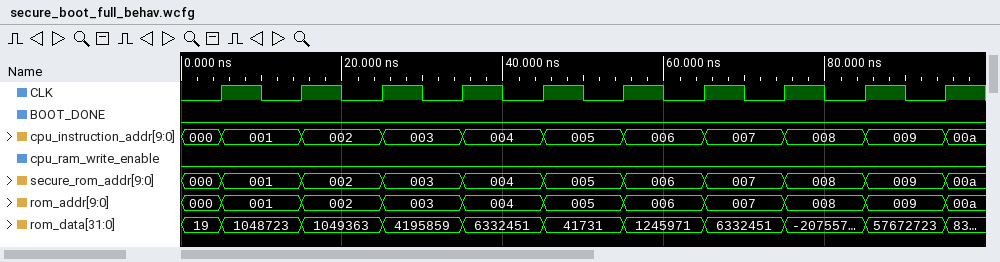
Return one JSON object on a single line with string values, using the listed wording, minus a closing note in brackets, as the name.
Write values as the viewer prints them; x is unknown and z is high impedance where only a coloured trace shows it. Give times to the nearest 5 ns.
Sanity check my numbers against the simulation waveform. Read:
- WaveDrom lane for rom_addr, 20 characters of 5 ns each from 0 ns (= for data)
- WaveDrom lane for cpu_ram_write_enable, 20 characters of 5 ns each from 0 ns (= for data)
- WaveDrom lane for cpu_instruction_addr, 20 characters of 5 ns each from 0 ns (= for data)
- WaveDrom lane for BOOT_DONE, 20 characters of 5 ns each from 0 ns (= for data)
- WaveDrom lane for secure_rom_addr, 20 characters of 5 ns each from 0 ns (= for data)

{"WaveDrom lane for rom_addr, 20 characters of 5 ns each from 0 ns": "{name: 'rom_addr', wave: '==.=.=.=.=.=.=.=.=.=', data: '000 001 002 003 004 005 006 007 008 009 00a'}", "WaveDrom lane for cpu_ram_write_enable, 20 characters of 5 ns each from 0 ns": "{name: 'cpu_ram_write_enable', wave: '0...................'}", "WaveDrom lane for cpu_instruction_addr, 20 characters of 5 ns each from 0 ns": "{name: 'cpu_instruction_addr', wave: '==.=.=.=.=.=.=.=.=.=', data: '000 001 002 003 004 005 006 007 008 009 00a'}", "WaveDrom lane for BOOT_DONE, 20 characters of 5 ns each from 0 ns": "{name: 'BOOT_DONE', wave: '0...................'}", "WaveDrom lane for secure_rom_addr, 20 characters of 5 ns each from 0 ns": "{name: 'secure_rom_addr', wave: '==.=.=.=.=.=.=.=.=.=', data: '000 001 002 003 004 005 006 007 008 009 00a'}"}
